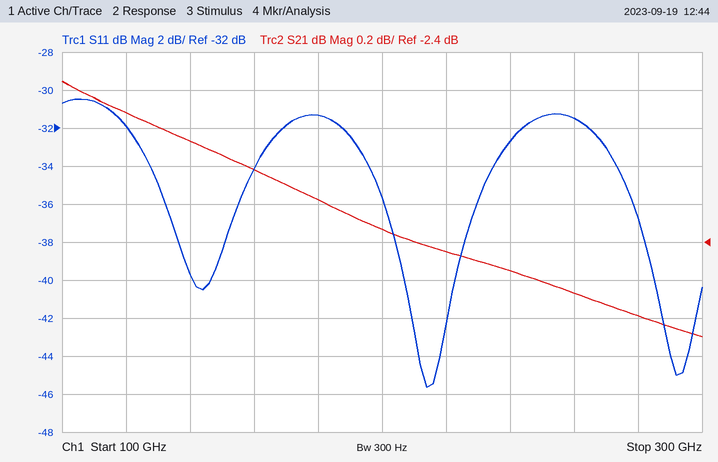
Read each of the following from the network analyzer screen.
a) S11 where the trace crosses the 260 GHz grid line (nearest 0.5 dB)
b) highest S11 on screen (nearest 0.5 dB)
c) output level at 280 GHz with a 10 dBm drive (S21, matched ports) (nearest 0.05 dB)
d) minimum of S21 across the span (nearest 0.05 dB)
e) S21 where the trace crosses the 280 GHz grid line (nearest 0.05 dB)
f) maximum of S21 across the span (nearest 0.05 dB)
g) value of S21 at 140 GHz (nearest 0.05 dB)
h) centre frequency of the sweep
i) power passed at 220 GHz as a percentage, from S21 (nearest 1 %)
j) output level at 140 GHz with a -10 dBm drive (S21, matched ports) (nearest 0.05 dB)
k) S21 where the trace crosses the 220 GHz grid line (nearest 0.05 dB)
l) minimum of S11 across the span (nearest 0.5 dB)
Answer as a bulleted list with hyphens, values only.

- -31.5 dB
- -30.5 dB
- 7.20 dBm
- -2.90 dB
- -2.80 dB
- -1.55 dB
- -1.85 dB
- 200 GHz
- 57 %
- -11.85 dBm
- -2.45 dB
- -45.5 dB
